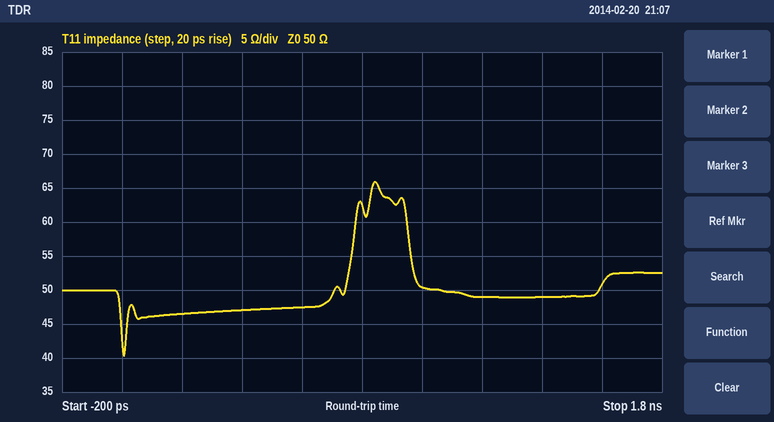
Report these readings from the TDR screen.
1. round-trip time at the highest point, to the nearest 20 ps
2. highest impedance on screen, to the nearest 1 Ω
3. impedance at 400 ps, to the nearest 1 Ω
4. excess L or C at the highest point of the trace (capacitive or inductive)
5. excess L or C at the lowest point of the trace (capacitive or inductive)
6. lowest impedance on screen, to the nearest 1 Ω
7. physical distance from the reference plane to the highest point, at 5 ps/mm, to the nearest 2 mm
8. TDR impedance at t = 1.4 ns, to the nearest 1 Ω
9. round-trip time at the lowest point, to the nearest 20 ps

840 ps
66 Ω
47 Ω
inductive
capacitive
40 Ω
84 mm
49 Ω
0 ps
